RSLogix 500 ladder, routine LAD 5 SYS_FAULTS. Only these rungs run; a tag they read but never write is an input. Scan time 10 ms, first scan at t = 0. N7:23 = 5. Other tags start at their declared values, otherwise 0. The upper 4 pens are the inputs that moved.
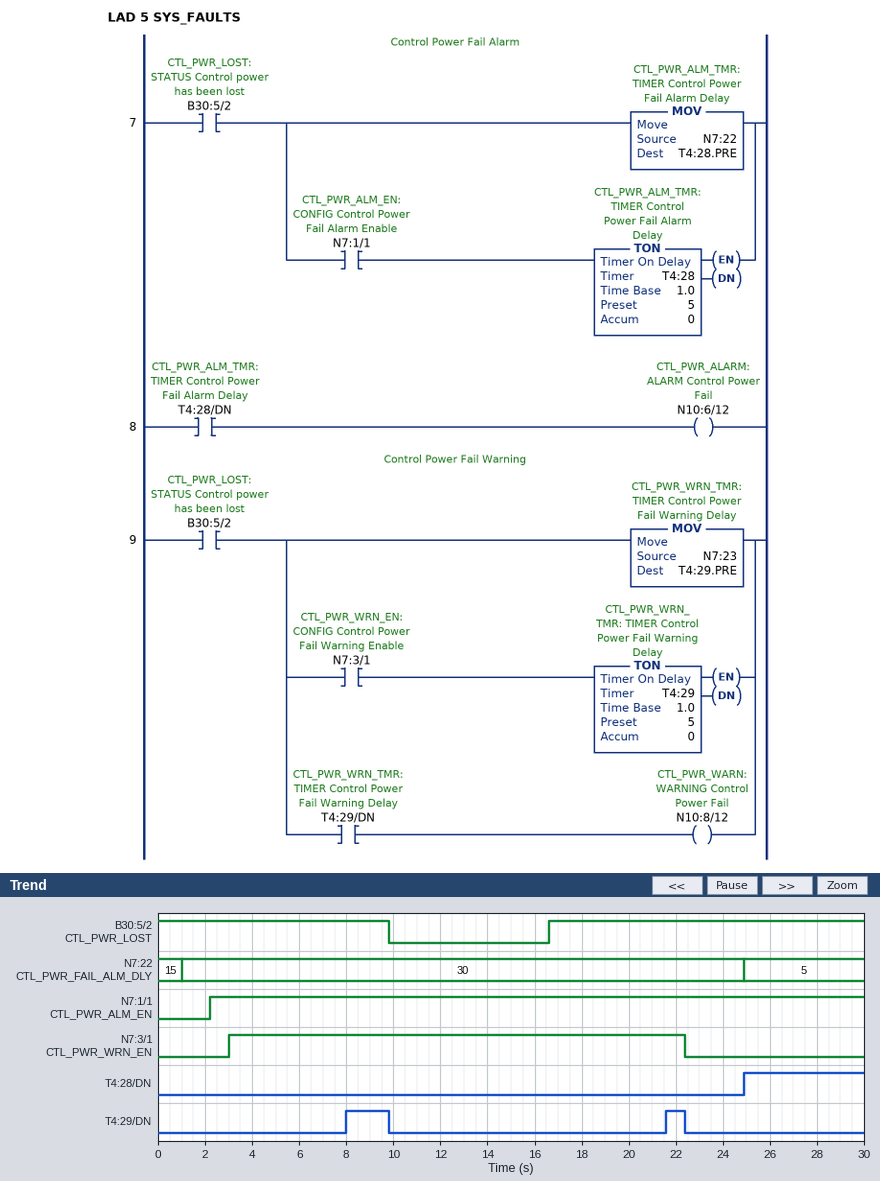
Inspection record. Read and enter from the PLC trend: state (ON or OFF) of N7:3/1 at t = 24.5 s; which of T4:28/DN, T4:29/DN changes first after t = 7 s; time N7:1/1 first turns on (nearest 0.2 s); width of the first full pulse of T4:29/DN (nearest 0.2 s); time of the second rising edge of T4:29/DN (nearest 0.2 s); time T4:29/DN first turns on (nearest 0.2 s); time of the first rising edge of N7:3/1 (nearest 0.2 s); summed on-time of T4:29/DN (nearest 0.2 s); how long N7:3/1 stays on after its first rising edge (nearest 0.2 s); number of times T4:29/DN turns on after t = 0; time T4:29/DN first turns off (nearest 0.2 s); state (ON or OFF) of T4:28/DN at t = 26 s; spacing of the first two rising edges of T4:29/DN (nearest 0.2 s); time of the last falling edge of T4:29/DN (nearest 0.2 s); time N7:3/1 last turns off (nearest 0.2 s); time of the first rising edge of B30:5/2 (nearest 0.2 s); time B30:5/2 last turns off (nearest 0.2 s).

OFF
T4:29/DN
2.2 s
1.8 s
21.6 s
8.0 s
3.0 s
2.6 s
19.4 s
2
9.8 s
ON
13.6 s
22.4 s
22.4 s
16.6 s
9.8 s
